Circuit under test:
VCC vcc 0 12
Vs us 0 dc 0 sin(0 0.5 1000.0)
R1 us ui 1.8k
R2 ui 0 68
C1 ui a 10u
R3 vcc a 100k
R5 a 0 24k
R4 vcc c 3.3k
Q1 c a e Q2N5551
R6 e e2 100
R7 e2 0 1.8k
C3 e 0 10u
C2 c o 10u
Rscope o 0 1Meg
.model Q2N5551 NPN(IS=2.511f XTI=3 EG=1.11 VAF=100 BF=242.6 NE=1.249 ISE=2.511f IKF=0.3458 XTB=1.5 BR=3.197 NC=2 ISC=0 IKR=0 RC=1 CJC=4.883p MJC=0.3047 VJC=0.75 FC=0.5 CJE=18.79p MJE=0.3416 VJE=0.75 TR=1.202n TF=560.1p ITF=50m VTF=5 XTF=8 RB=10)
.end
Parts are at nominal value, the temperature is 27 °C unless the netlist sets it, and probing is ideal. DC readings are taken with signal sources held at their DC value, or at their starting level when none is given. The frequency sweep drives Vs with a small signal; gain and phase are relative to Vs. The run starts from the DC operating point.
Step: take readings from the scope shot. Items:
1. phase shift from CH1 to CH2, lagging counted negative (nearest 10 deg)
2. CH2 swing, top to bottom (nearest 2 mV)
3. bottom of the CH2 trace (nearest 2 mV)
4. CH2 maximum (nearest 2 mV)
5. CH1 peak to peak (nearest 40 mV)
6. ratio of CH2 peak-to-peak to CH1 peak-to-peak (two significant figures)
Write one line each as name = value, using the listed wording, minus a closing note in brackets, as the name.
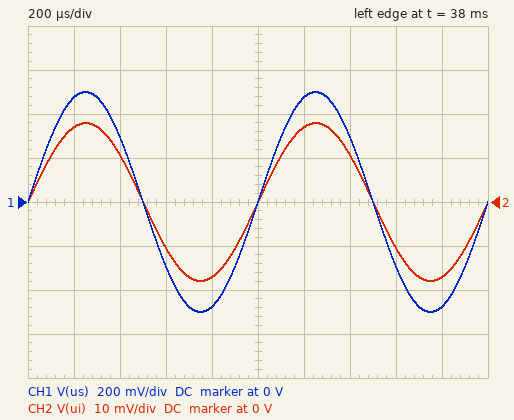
phase shift from CH1 to CH2, lagging counted negative = 0 deg
CH2 swing, top to bottom = 36 mV
bottom of the CH2 trace = -18 mV
CH2 maximum = 18 mV
CH1 peak to peak = 1.00 V
ratio of CH2 peak-to-peak to CH1 peak-to-peak = 0.036
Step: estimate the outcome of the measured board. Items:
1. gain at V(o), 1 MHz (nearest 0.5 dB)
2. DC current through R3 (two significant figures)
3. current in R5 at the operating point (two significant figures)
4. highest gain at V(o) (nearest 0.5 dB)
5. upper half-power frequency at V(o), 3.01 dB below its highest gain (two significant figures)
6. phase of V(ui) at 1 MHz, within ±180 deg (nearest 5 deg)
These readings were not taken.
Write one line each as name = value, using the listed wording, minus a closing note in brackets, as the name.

gain at V(o), 1 MHz = 10.5 dB
DC current through R3 = 98 µA
current in R5 at the operating point = 91 µA
highest gain at V(o) = 11.0 dB
upper half-power frequency at V(o), 3.01 dB below its highest gain = 5.8 MHz
phase of V(ui) at 1 MHz, within ±180 deg = -5 deg
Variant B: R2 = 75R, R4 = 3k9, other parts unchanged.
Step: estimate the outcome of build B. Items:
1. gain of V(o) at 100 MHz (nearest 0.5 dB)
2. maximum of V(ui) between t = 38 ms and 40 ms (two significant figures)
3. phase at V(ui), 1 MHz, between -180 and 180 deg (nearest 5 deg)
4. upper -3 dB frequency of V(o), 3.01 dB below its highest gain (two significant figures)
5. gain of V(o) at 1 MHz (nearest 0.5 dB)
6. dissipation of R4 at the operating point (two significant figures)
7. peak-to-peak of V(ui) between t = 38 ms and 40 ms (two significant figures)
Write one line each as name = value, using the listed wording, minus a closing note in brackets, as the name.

gain of V(o) at 100 MHz = -15.0 dB
maximum of V(ui) between t = 38 ms and 40 ms = 20 mV
phase at V(ui), 1 MHz, between -180 and 180 deg = -10 deg
upper -3 dB frequency of V(o), 3.01 dB below its highest gain = 4.6 MHz
gain of V(o) at 1 MHz = 13.0 dB
dissipation of R4 at the operating point = 2.4 mW
peak-to-peak of V(ui) between t = 38 ms and 40 ms = 39 mV
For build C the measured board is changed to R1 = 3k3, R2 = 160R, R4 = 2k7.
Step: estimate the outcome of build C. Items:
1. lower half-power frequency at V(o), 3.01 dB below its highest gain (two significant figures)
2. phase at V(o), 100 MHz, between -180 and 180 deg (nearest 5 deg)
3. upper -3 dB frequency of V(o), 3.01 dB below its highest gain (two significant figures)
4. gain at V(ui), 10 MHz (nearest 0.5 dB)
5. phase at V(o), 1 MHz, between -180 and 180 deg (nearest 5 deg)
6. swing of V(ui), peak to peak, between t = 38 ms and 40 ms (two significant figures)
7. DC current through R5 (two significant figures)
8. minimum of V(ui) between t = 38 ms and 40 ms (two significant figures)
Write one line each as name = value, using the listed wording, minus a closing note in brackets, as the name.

lower half-power frequency at V(o), 3.01 dB below its highest gain = 470 Hz
phase at V(o), 100 MHz, between -180 and 180 deg = 55 deg
upper -3 dB frequency of V(o), 3.01 dB below its highest gain = 3.8 MHz
gain at V(ui), 10 MHz = -35.0 dB
phase at V(o), 1 MHz, between -180 and 180 deg = 165 deg
swing of V(ui), peak to peak, between t = 38 ms and 40 ms = 45 mV
DC current through R5 = 91 µA
minimum of V(ui) between t = 38 ms and 40 ms = -22 mV
